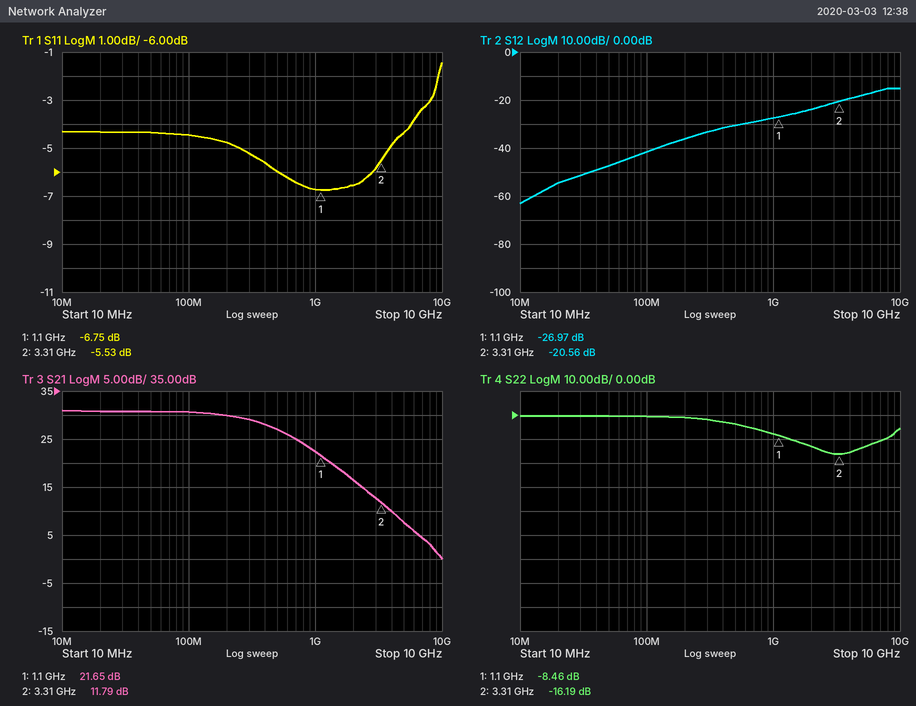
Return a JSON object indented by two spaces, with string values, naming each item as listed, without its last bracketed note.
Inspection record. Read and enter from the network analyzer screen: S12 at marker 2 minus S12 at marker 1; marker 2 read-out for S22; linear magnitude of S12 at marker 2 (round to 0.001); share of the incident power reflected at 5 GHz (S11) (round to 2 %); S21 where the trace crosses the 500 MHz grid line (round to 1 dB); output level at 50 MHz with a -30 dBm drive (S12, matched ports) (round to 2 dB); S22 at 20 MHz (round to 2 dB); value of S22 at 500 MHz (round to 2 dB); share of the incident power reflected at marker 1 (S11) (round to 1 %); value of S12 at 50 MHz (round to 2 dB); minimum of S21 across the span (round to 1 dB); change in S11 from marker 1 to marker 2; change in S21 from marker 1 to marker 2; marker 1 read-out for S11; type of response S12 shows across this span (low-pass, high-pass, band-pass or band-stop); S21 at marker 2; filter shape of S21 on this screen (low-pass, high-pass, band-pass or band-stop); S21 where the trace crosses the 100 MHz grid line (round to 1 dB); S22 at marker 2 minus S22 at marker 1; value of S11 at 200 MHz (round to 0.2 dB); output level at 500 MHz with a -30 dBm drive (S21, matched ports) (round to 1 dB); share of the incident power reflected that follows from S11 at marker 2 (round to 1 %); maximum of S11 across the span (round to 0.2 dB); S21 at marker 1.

{
  "S12 at marker 2 minus S12 at marker 1": "6.41 dB",
  "marker 2 read-out for S22": "-16.19 dB",
  "linear magnitude of S12 at marker 2": "0.094",
  "share of the incident power reflected at 5 GHz (S11)": "36 %",
  "S21 where the trace crosses the 500 MHz grid line": "27 dB",
  "output level at 50 MHz with a -30 dBm drive (S12, matched ports)": "-78 dBm",
  "S22 at 20 MHz": "0 dB",
  "value of S22 at 500 MHz": "-4 dB",
  "share of the incident power reflected at marker 1 (S11)": "21 %",
  "value of S12 at 50 MHz": "-48 dB",
  "minimum of S21 across the span": "0 dB",
  "change in S11 from marker 1 to marker 2": "1.22 dB",
  "change in S21 from marker 1 to marker 2": "-9.86 dB",
  "marker 1 read-out for S11": "-6.75 dB",
  "type of response S12 shows across this span": "high-pass",
  "S21 at marker 2": "11.79 dB",
  "filter shape of S21 on this screen": "low-pass",
  "S21 where the trace crosses the 100 MHz grid line": "31 dB",
  "S22 at marker 2 minus S22 at marker 1": "-7.73 dB",
  "value of S11 at 200 MHz": "-4.8 dB",
  "output level at 500 MHz with a -30 dBm drive (S21, matched ports)": "-3 dBm",
  "share of the incident power reflected that follows from S11 at marker 2": "28 %",
  "maximum of S11 across the span": "-1.4 dB",
  "S21 at marker 1": "21.65 dB"
}
